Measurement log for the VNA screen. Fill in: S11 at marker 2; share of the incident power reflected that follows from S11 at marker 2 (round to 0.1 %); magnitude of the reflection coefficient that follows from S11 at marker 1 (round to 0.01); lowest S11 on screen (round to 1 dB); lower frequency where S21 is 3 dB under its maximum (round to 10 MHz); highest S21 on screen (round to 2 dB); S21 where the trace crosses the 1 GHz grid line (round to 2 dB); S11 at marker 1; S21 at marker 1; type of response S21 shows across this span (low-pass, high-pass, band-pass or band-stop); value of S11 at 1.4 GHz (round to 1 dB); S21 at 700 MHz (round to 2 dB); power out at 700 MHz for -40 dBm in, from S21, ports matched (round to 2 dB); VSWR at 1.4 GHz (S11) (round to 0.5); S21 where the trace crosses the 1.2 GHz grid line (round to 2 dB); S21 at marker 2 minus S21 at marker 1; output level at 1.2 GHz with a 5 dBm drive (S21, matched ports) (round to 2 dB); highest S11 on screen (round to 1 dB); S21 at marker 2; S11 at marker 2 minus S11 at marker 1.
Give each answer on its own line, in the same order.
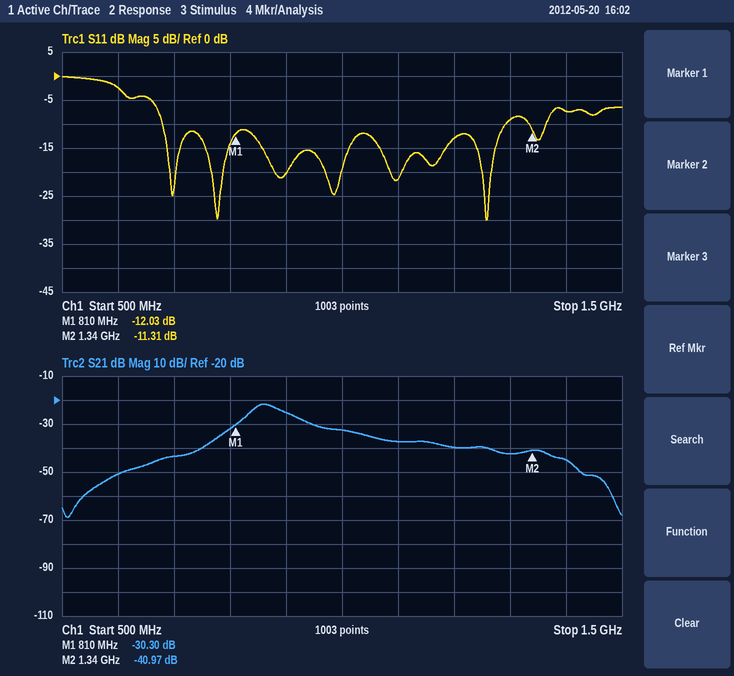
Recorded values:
-11.31 dB
7.4 %
0.25
-30 dB
840 MHz
-22 dB
-32 dB
-12.03 dB
-30.30 dB
band-pass
-7 dB
-44 dB
-84 dBm
2.5
-40 dB
-10.67 dB
-34 dBm
0 dB
-40.97 dB
0.72 dB
